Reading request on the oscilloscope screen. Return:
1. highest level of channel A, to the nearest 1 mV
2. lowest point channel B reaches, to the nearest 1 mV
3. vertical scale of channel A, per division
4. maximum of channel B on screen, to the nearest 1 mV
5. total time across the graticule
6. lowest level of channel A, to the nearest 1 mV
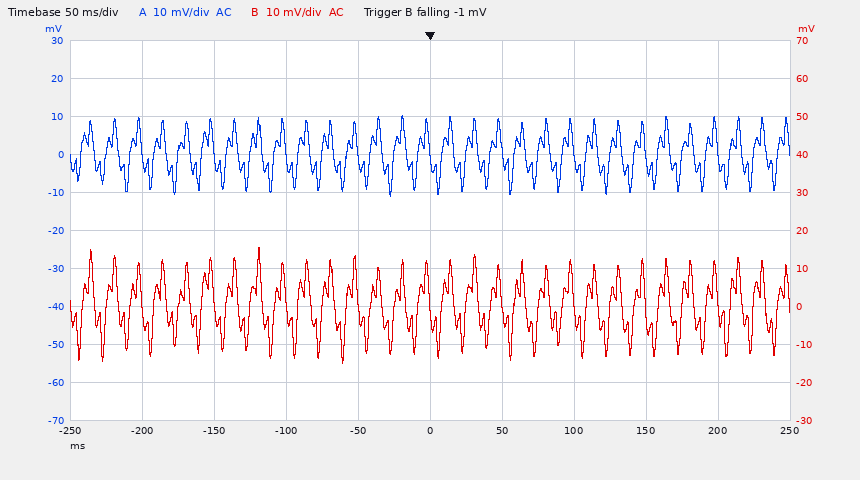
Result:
10 mV
-15 mV
10 mV
16 mV
500 ms
-11 mV
